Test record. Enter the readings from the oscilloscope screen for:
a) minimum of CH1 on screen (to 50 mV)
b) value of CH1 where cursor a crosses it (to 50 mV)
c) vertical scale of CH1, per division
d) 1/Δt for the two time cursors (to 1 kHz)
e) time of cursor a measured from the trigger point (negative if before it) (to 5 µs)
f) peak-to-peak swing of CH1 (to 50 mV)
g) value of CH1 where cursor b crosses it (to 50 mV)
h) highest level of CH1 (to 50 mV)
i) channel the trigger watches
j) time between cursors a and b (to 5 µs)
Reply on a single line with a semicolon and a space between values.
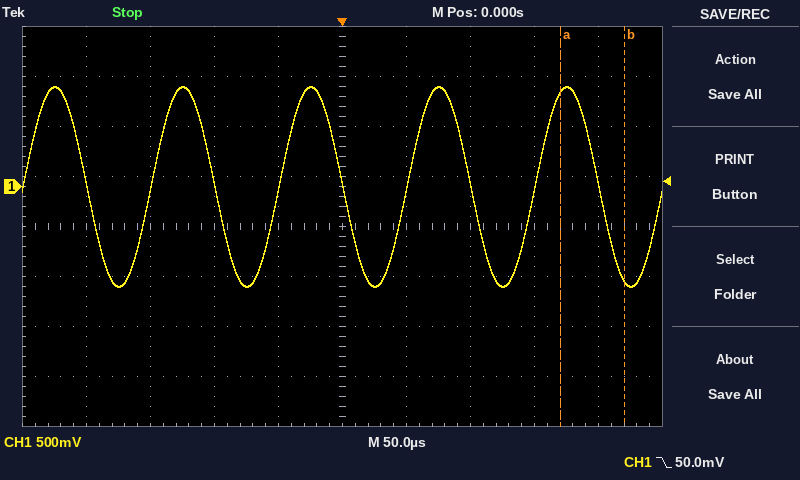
-1.00 V; 950 mV; 500 mV; 20 kHz; +170 µs; 2.00 V; -950 mV; 1.00 V; CH1; 50 µs
